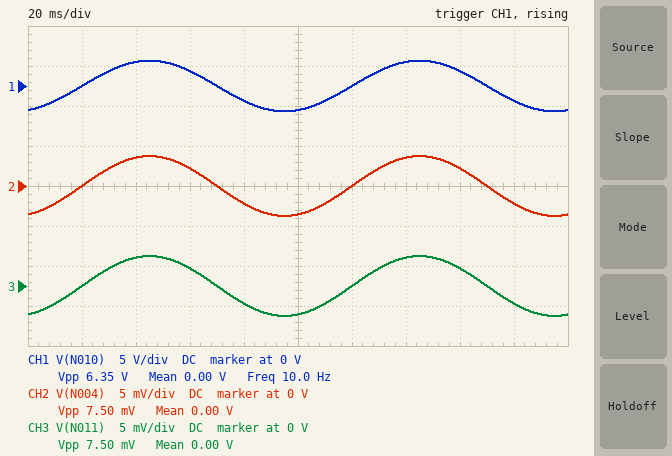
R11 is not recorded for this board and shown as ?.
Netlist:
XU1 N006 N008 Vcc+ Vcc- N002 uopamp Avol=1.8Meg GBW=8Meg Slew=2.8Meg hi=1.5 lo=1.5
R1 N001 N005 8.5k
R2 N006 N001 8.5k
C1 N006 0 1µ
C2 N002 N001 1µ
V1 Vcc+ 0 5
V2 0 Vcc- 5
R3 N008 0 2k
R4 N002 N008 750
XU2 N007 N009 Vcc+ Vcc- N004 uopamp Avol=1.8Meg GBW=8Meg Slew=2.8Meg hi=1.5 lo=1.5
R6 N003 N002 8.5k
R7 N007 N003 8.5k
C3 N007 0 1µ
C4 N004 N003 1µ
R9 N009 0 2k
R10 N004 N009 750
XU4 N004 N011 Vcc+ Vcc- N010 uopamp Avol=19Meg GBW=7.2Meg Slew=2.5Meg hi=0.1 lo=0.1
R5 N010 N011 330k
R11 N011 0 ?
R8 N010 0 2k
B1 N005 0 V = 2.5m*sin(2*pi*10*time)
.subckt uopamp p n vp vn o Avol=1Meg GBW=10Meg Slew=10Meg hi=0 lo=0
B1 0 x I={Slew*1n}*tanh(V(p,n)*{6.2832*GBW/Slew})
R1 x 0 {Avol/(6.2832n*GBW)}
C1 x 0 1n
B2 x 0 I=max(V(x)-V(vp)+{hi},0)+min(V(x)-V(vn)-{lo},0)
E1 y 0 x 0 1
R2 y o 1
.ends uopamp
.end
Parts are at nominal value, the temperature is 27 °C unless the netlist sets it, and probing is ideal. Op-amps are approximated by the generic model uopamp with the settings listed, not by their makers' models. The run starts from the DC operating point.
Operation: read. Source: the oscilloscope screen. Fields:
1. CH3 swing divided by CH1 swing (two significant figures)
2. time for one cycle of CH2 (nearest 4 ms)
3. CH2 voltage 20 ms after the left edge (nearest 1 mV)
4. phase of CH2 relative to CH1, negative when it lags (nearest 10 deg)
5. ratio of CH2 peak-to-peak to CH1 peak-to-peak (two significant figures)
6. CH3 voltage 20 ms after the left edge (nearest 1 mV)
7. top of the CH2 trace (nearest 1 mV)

0.0012
100 ms
0 V
0 deg
0.0012
0 V
4 mV
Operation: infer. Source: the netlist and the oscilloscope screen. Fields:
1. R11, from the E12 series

390 Ω
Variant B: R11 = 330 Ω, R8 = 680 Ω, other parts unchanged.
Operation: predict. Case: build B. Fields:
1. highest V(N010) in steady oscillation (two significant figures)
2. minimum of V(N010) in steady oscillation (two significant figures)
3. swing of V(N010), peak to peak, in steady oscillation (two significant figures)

3.7 V
-3.7 V
7.5 V
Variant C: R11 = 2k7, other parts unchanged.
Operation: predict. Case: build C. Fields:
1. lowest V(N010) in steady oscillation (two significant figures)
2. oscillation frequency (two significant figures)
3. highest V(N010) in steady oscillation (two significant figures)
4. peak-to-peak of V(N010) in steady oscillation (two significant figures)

-460 mV
10 Hz
460 mV
920 mV
